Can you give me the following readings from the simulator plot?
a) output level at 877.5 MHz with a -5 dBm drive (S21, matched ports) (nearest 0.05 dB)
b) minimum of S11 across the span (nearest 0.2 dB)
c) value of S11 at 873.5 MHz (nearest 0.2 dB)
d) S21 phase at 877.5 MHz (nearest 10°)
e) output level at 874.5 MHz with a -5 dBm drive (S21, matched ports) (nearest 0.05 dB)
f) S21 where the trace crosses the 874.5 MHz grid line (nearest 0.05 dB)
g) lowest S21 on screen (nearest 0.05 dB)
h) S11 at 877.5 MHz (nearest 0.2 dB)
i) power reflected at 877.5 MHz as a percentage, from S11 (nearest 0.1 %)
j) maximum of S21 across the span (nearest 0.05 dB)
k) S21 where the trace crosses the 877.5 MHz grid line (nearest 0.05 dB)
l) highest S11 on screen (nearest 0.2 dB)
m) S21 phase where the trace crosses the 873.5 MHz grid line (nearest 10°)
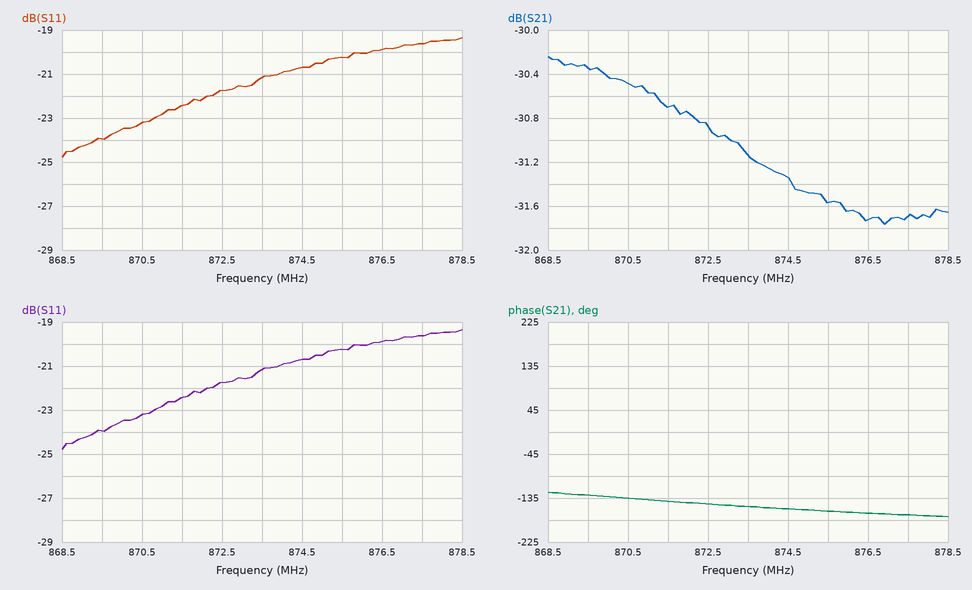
-36.70 dBm
-24.8 dB
-21.2 dB
-170°
-36.35 dBm
-31.35 dB
-31.75 dB
-19.6 dB
1.1 %
-30.25 dB
-31.70 dB
-19.4 dB
-150°
